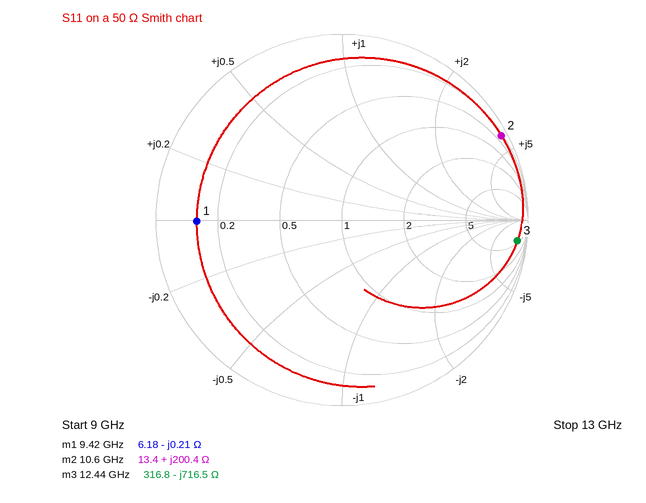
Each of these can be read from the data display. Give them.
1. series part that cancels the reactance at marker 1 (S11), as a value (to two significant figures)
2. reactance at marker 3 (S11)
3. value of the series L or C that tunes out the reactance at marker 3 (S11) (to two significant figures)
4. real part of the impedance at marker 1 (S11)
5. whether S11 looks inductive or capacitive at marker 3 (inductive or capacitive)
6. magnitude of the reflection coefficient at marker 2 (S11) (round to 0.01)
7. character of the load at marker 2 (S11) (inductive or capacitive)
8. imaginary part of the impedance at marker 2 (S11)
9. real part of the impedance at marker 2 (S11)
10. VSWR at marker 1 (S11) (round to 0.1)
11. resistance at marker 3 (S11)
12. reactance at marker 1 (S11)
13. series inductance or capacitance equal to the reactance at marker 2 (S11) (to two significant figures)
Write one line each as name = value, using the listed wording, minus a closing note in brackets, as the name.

series part that cancels the reactance at marker 1 (S11), as a value = 3.5 pH
reactance at marker 3 = -716.5 Ω
value of the series L or C that tunes out the reactance at marker 3 (S11) = 9.2 nH
real part of the impedance at marker 1 = 6.18 Ω
whether S11 looks inductive or capacitive at marker 3 = capacitive
magnitude of the reflection coefficient at marker 2 (S11) = 0.97
character of the load at marker 2 (S11) = inductive
imaginary part of the impedance at marker 2 = +200.4 Ω
real part of the impedance at marker 2 = 13.4 Ω
VSWR at marker 1 (S11) = 8.1
resistance at marker 3 = 316.8 Ω
reactance at marker 1 = -0.21 Ω
series inductance or capacitance equal to the reactance at marker 2 (S11) = 3.0 nH
